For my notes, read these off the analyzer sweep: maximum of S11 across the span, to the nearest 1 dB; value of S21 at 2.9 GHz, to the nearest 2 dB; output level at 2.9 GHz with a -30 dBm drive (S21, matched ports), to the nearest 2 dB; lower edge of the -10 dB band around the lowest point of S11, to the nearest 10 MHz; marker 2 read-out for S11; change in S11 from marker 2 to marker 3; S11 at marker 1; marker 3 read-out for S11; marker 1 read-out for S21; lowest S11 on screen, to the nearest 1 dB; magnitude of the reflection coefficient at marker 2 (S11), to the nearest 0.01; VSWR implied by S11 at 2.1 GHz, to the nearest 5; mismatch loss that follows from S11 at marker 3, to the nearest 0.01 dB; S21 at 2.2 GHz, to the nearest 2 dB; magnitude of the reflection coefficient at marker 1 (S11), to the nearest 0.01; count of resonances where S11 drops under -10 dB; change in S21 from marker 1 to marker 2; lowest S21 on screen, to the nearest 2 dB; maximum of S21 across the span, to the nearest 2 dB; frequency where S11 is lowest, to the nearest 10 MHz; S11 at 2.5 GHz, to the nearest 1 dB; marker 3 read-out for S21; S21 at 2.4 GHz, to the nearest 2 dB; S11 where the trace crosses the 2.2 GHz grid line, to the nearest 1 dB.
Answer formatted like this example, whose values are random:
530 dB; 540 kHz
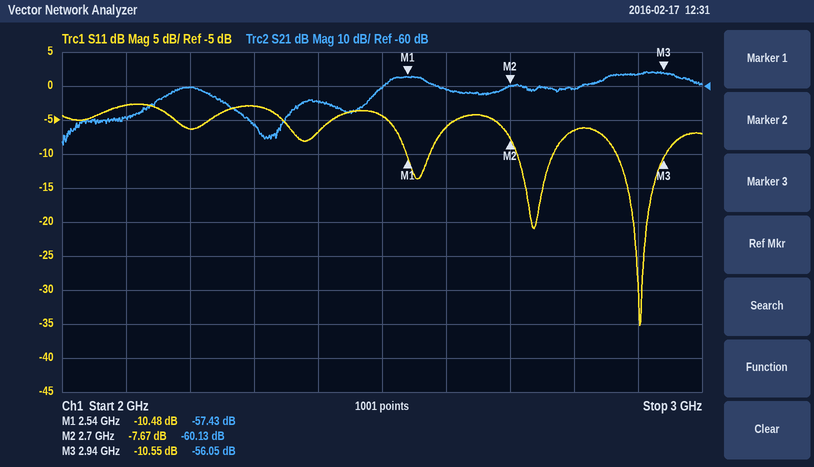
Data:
-3 dB; -56 dB; -86 dBm; 2.87 GHz; -7.67 dB; -2.88 dB; -10.48 dB; -10.55 dB; -57.43 dB; -35 dB; 0.41; 5; 0.40 dB; -60 dB; 0.30; 3; -2.70 dB; -78 dB; -56 dB; 2.90 GHz; -4 dB; -56.05 dB; -64 dB; -6 dB
